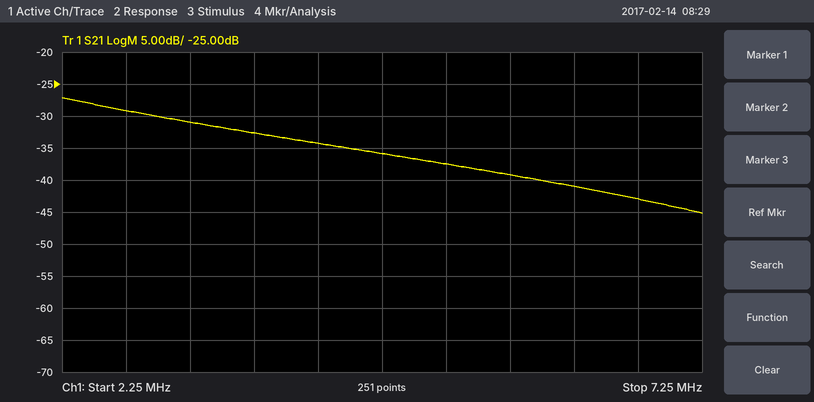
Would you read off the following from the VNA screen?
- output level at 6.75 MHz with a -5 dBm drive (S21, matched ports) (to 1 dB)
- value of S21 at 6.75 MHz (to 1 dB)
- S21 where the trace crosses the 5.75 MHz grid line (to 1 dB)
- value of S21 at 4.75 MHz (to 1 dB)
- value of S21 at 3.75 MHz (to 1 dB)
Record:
-48 dBm
-43 dB
-39 dB
-36 dB
-33 dB
